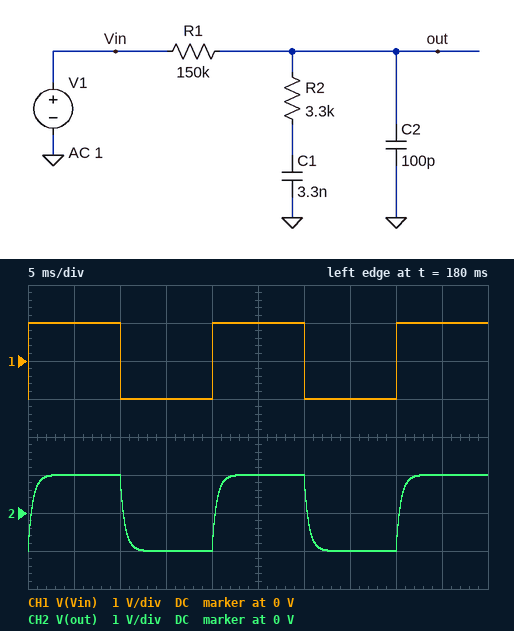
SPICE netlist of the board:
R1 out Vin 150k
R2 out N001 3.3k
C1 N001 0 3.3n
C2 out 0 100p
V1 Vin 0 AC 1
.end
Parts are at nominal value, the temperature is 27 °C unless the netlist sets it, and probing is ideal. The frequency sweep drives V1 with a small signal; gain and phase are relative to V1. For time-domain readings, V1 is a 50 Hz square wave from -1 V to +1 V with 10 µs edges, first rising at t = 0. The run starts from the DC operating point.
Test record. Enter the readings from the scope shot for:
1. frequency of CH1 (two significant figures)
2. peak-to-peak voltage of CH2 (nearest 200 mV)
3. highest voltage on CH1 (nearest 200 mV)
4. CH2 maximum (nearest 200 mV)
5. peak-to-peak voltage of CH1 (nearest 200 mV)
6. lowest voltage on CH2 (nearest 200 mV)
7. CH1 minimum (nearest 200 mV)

50 Hz
2.0 V
1.0 V
1.0 V
2.0 V
-1.0 V
-1.0 V
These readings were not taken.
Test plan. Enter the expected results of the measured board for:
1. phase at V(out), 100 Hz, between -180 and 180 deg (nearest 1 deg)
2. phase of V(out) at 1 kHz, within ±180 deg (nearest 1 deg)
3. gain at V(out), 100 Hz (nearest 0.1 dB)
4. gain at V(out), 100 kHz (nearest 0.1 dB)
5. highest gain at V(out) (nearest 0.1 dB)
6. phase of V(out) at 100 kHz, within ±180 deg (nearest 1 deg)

-18 deg
-69 deg
-0.4 dB
-33.7 dB
0 dB
-19 deg
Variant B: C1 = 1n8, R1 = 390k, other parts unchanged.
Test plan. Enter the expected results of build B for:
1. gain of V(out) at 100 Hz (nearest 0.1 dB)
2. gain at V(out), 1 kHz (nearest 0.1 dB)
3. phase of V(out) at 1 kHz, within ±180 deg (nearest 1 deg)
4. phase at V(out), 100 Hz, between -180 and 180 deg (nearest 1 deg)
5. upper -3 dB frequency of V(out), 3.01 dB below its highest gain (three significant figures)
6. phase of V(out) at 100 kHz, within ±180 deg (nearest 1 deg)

-0.9 dB
-13.6 dB
-76 deg
-25 deg
213 Hz
-26 deg
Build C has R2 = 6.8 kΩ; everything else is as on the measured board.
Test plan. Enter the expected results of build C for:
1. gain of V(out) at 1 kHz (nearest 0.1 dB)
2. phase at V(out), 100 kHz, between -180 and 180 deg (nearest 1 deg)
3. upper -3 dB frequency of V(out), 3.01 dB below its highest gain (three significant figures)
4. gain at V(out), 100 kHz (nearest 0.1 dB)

-10.8 dB
-26 deg
300 Hz
-28.1 dB
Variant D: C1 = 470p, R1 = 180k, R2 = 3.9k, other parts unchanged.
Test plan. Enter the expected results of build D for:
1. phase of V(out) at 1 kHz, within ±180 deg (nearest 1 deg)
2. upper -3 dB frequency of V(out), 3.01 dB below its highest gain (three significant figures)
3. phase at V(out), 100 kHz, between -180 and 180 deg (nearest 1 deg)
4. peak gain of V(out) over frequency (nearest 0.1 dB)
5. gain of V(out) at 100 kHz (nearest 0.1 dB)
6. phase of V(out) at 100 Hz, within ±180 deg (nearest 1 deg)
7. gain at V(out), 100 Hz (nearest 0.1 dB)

-33 deg
1.53 kHz
-51 deg
0 dB
-32.8 dB
-4 deg
0 dB
